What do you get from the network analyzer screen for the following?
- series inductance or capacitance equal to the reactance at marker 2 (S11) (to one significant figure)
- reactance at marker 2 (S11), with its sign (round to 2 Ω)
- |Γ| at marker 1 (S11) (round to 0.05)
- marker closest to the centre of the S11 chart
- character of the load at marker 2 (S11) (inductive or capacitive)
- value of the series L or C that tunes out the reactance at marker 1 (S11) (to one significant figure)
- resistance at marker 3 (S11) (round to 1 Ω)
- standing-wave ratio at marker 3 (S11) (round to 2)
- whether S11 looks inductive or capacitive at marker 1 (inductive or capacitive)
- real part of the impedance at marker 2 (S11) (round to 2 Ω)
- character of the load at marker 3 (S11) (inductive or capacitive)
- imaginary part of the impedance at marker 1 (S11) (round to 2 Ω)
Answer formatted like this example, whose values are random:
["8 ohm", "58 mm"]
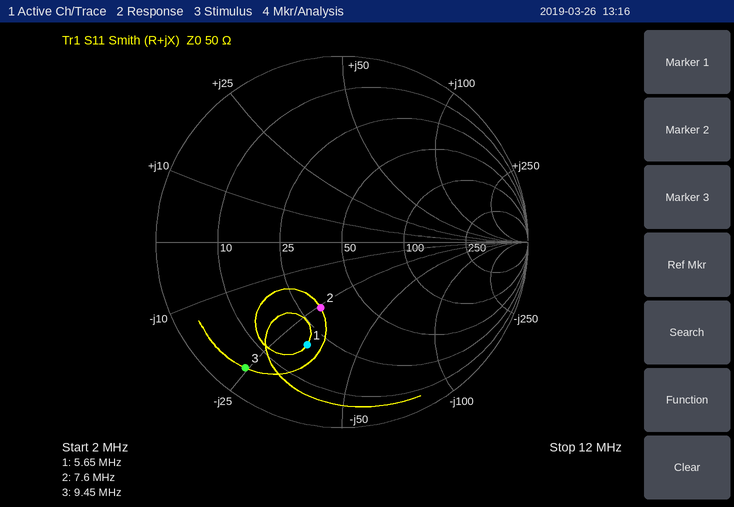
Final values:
["800 pF", "-26 Ω", "0.60", "marker 2", "capacitive", "900 nH", "5 Ω", "12", "capacitive", "32 Ω", "capacitive", "-32 Ω"]
